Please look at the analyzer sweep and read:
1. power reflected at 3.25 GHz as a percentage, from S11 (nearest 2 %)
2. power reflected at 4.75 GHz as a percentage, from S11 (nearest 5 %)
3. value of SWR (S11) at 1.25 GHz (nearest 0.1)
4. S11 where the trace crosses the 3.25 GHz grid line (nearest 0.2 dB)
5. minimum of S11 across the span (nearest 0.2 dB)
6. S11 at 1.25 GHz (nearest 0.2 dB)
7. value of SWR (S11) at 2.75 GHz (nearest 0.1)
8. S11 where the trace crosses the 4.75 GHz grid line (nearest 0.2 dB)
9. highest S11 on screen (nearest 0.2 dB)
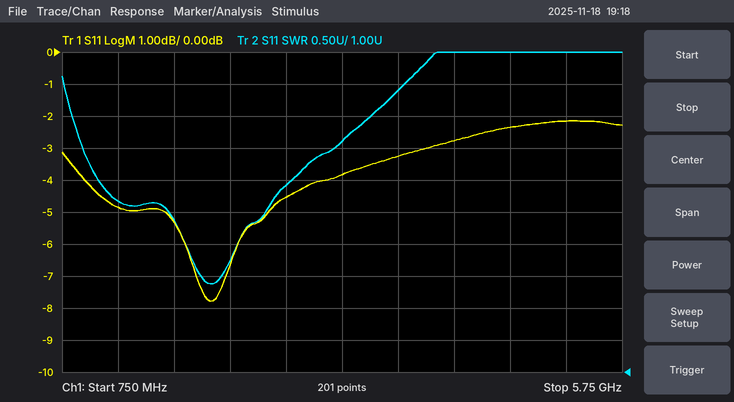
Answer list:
42 %
60 %
3.7
-3.8 dB
-7.8 dB
-4.8 dB
3.9
-2.4 dB
-2.2 dB
